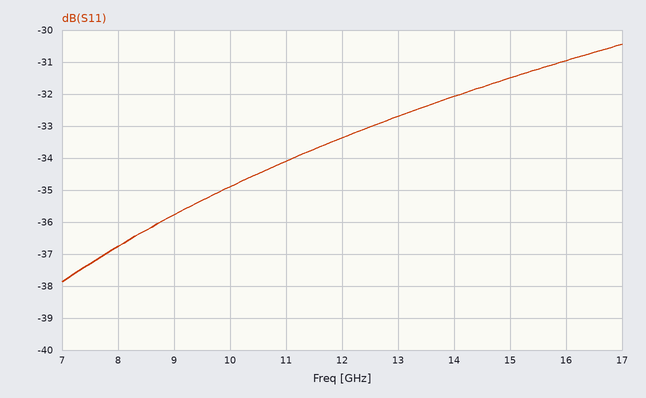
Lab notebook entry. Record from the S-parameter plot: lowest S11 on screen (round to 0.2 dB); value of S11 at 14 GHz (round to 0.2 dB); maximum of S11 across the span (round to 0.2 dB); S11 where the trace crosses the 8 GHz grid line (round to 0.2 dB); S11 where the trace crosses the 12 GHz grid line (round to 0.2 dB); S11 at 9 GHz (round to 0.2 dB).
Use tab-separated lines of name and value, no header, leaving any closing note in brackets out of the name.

lowest S11 on screen	-37.8 dB
value of S11 at 14 GHz	-32.0 dB
maximum of S11 across the span	-30.4 dB
S11 where the trace crosses the 8 GHz grid line	-36.8 dB
S11 where the trace crosses the 12 GHz grid line	-33.4 dB
S11 at 9 GHz	-35.8 dB
